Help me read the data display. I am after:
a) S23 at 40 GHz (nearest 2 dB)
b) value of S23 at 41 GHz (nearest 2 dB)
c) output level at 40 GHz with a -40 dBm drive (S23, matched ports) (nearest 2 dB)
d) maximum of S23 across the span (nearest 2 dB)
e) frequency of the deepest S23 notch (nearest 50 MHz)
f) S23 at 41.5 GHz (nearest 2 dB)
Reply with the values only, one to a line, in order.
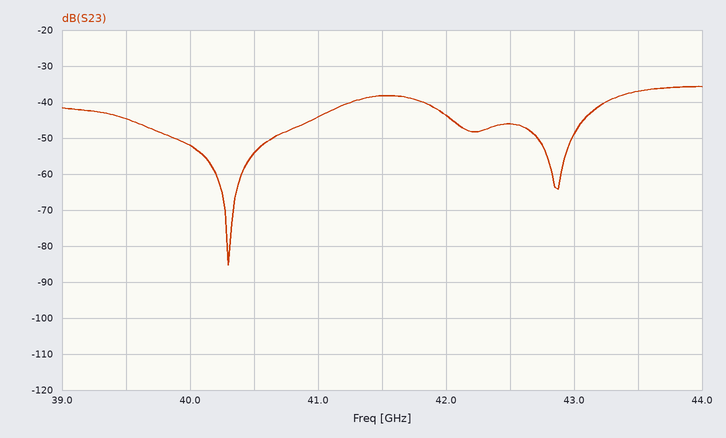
-52 dB
-44 dB
-92 dBm
-36 dB
40.30 GHz
-38 dB
